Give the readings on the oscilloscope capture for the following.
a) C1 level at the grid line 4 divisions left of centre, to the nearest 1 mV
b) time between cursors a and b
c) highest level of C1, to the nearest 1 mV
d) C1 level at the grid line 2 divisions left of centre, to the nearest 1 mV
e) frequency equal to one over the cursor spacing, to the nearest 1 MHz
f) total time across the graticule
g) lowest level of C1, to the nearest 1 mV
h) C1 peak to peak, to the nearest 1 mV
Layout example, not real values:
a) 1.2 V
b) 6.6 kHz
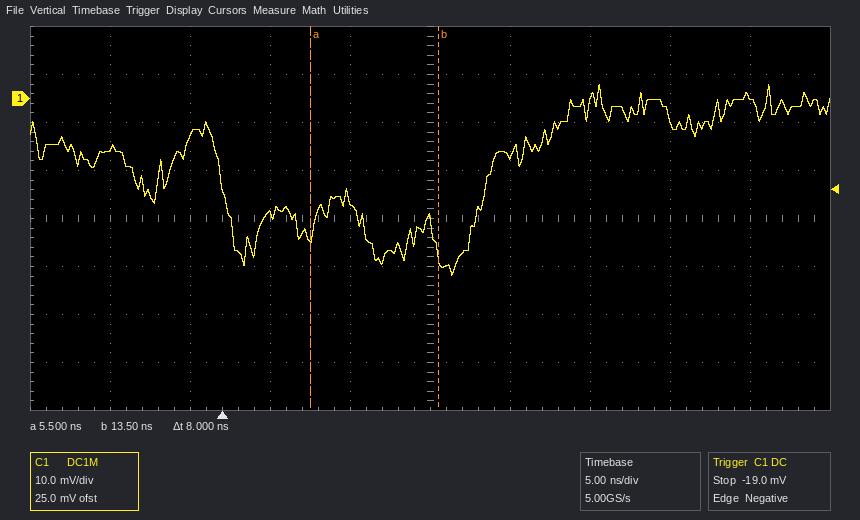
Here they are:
a) -10 mV
b) 8 ns
c) 3 mV
d) -24 mV
e) 125 MHz
f) 50 ns
g) -37 mV
h) 40 mV
